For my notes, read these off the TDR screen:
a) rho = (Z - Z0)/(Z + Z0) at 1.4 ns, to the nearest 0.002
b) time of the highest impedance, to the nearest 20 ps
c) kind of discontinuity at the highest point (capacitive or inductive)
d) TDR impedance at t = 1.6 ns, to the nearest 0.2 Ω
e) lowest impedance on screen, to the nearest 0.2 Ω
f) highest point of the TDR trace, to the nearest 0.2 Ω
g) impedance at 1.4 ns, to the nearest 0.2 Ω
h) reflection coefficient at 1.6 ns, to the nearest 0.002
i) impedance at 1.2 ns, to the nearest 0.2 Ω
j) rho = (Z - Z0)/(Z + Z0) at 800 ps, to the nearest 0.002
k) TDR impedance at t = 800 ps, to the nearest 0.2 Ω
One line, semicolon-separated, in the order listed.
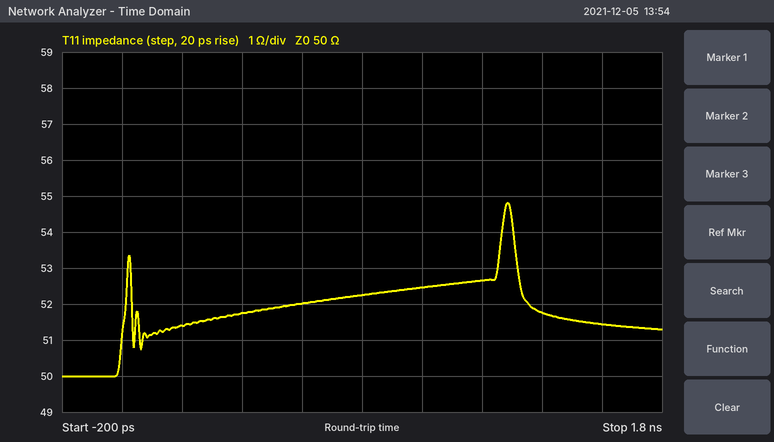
+0.018; 1.28 ns; inductive; 51.4 Ω; 50.0 Ω; 54.8 Ω; 51.8 Ω; +0.014; 52.6 Ω; +0.022; 52.2 Ω
